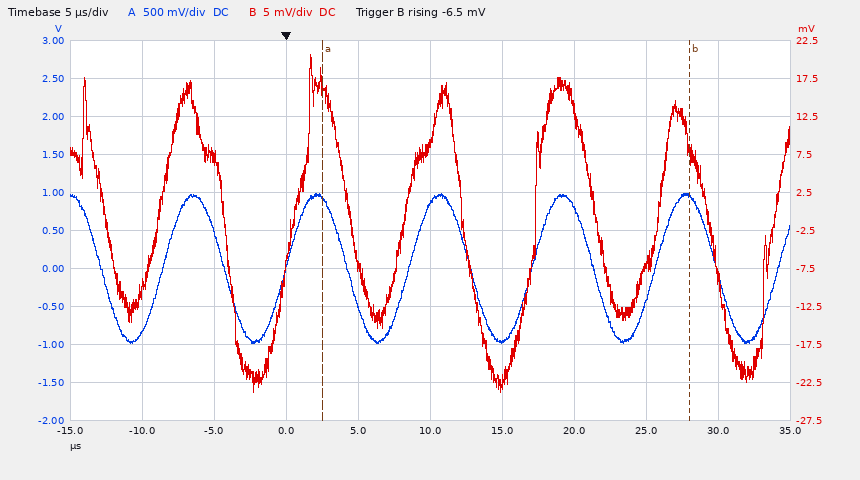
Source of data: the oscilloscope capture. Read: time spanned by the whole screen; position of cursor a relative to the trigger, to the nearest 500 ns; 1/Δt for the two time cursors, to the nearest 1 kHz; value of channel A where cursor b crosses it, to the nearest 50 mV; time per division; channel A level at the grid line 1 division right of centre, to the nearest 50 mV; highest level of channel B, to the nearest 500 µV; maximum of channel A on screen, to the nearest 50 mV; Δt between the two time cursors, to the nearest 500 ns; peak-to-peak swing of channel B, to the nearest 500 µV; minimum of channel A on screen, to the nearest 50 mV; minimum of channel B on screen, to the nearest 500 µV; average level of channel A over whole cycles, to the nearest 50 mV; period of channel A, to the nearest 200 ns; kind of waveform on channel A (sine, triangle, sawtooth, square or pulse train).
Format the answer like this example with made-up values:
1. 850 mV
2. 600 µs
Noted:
1. 50 µs
2. +2.5 µs
3. 39 kHz
4. 950 mV
5. 5 µs
6. -950 mV
7. 20.5 mV
8. 1.00 V
9. 25.5 µs
10. 44.5 mV
11. -1.00 V
12. -24.0 mV
13. 0 mV
14. 8.6 µs
15. sine
